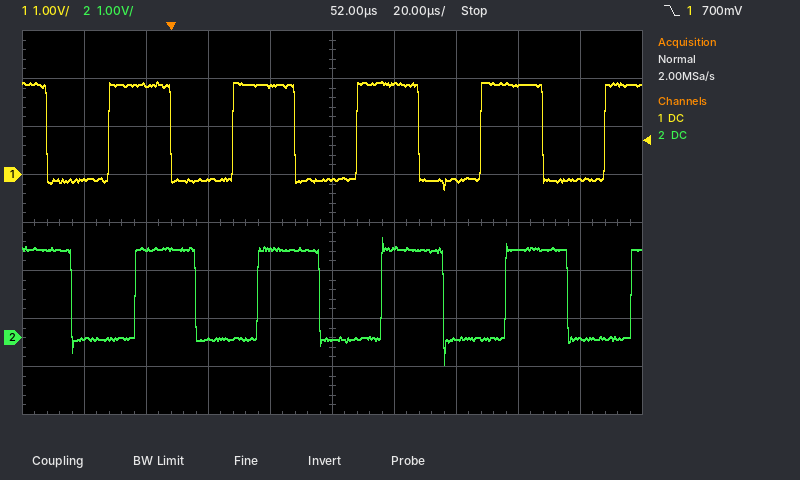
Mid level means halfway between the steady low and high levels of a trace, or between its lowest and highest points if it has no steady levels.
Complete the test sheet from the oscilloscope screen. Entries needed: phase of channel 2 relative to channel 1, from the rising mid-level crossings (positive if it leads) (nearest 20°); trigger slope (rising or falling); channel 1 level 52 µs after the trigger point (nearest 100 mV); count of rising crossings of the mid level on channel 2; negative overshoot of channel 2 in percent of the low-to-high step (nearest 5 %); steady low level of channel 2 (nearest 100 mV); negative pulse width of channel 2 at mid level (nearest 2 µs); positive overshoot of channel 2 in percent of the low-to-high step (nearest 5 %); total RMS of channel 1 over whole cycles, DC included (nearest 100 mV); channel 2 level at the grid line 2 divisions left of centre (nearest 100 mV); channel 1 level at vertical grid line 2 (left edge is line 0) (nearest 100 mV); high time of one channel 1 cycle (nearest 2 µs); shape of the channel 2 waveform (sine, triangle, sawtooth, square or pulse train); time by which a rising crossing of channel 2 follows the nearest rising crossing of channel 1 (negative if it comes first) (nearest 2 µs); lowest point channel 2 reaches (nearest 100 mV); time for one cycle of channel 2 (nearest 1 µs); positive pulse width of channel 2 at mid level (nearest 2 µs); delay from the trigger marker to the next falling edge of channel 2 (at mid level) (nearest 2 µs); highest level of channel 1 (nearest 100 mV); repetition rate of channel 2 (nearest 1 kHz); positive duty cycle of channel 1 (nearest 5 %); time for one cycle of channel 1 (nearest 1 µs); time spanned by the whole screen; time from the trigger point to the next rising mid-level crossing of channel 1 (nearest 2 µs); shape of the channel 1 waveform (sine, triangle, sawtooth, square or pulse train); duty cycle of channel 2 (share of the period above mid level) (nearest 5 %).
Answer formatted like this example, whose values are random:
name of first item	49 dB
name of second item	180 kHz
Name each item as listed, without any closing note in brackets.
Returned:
phase of channel 2 relative to channel 1, from the rising mid-level crossings (positive if it leads)	-80°
trigger slope	falling
channel 1 level 52 µs after the trigger point	-100 mV
count of rising crossings of the mid level on channel 2	5
negative overshoot of channel 2 in percent of the low-to-high step	30 %
steady low level of channel 2	0.0 V
negative pulse width of channel 2 at mid level	20 µs
positive overshoot of channel 2 in percent of the low-to-high step	15 %
total RMS of channel 1 over whole cycles, DC included	1.3 V
channel 2 level at the grid line 2 divisions left of centre	0.0 V
channel 1 level at vertical grid line 2 (left edge is line 0)	1.9 V
high time of one channel 1 cycle	20 µs
shape of the channel 2 waveform	square
time by which a rising crossing of channel 2 follows the nearest rising crossing of channel 1 (negative if it comes first)	+8 µs
lowest point channel 2 reaches	-600 mV
time for one cycle of channel 2	40 µs
positive pulse width of channel 2 at mid level	20 µs
delay from the trigger marker to the next falling edge of channel 2 (at mid level)	8 µs
highest level of channel 1	1.9 V
repetition rate of channel 2	25 kHz
positive duty cycle of channel 1	50 %
time for one cycle of channel 1	40 µs
time spanned by the whole screen	200 µs
time from the trigger point to the next rising mid-level crossing of channel 1	20 µs
shape of the channel 1 waveform	square
duty cycle of channel 2 (share of the period above mid level)	50 %
